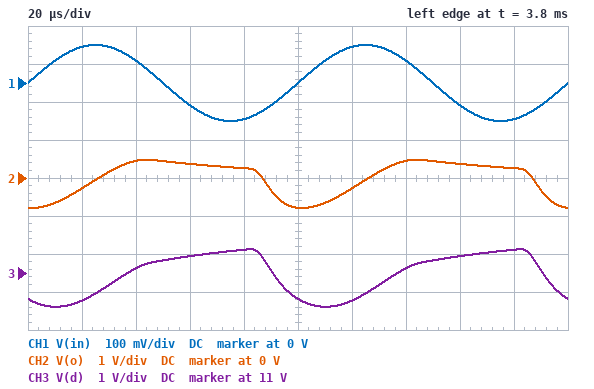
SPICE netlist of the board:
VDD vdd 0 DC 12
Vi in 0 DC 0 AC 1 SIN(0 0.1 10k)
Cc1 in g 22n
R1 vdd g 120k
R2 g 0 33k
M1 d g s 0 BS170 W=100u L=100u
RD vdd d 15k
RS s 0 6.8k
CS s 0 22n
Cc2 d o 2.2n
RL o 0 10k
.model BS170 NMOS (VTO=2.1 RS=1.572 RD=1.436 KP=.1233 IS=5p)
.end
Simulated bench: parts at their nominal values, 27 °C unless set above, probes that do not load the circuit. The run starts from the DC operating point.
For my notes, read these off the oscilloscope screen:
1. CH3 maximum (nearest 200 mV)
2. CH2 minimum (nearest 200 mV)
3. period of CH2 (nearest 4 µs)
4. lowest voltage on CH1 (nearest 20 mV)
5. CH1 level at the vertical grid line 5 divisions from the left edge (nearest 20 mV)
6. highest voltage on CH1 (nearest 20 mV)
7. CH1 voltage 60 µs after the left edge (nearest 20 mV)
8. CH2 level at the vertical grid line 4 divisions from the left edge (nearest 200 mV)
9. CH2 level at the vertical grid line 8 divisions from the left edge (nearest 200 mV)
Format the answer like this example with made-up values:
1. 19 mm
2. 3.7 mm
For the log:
1. 11.6 V
2. -800 mV
3. 100 µs
4. -100 mV
5. 0 V
6. 100 mV
7. -60 mV
8. 200 mV
9. 400 mV
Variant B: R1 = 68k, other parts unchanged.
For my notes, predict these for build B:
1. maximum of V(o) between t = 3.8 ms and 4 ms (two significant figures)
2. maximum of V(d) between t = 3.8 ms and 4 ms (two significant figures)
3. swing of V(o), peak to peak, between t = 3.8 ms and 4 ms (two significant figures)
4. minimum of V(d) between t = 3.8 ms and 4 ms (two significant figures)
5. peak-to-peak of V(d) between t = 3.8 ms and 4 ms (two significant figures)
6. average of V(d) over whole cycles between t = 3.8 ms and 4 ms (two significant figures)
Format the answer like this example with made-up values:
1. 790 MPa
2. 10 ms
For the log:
1. 760 mV
2. 9.1 V
3. 1.5 V
4. 7.2 V
5. 1.9 V
6. 8.1 V
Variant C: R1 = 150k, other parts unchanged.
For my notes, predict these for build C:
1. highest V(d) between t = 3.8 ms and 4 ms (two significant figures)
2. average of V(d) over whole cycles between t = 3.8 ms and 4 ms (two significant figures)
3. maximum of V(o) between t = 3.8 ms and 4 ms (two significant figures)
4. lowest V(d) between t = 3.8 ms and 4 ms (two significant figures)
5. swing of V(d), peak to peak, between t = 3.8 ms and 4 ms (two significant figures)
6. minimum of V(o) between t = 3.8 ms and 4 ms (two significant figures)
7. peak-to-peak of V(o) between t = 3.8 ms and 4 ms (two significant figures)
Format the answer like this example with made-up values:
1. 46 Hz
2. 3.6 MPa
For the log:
1. 12 V
2. 12 V
3. 150 mV
4. 11 V
5. 650 mV
6. -460 mV
7. 610 mV
